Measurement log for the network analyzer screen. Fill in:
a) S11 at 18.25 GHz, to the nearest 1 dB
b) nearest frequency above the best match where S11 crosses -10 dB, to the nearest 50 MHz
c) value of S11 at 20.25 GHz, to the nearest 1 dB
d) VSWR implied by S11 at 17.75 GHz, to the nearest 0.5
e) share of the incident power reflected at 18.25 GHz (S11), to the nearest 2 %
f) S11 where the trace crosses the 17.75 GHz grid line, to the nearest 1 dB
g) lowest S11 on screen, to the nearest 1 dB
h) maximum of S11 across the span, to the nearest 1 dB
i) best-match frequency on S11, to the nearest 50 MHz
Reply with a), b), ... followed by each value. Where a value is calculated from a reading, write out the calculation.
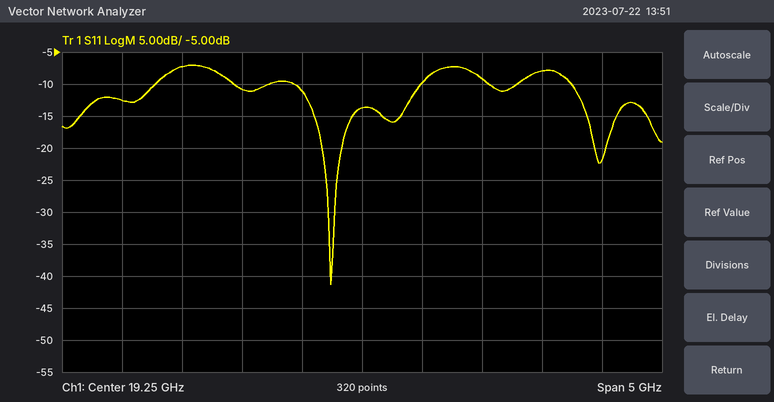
a) -11 dB
b) 19.75 GHz
c) -9 dB
d) |Γ| = 10^(-7/20) = 0.4467; VSWR = (1 + 0.4467)/(1 − 0.4467) ≈ 2.61, so 2.5 to the nearest 0.5
e) 10^(-11/10) ≈ 8 %
f) -7 dB
g) -41 dB
h) -7 dB
i) 19.00 GHz
